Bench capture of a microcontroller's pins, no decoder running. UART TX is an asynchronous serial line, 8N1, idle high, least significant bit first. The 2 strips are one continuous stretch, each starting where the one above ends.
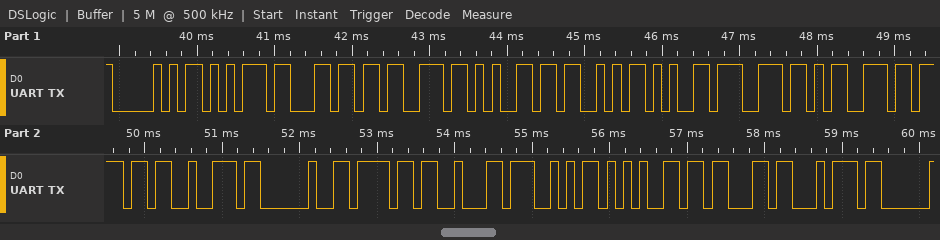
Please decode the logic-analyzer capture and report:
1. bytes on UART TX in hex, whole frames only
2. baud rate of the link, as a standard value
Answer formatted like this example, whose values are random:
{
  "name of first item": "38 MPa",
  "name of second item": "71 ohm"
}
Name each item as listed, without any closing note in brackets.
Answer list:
{
  "bytes on UART TX in hex, whole frames only": "0x50 0x75 0x6C 0x73 0x65 0x53 0x65 0x6E 0x73 0x6F 0x72 0x20 0x6F 0x62 0x6A 0x65 0x63 0x74",
  "baud rate of the link, as a standard value": "9600 baud"
}
